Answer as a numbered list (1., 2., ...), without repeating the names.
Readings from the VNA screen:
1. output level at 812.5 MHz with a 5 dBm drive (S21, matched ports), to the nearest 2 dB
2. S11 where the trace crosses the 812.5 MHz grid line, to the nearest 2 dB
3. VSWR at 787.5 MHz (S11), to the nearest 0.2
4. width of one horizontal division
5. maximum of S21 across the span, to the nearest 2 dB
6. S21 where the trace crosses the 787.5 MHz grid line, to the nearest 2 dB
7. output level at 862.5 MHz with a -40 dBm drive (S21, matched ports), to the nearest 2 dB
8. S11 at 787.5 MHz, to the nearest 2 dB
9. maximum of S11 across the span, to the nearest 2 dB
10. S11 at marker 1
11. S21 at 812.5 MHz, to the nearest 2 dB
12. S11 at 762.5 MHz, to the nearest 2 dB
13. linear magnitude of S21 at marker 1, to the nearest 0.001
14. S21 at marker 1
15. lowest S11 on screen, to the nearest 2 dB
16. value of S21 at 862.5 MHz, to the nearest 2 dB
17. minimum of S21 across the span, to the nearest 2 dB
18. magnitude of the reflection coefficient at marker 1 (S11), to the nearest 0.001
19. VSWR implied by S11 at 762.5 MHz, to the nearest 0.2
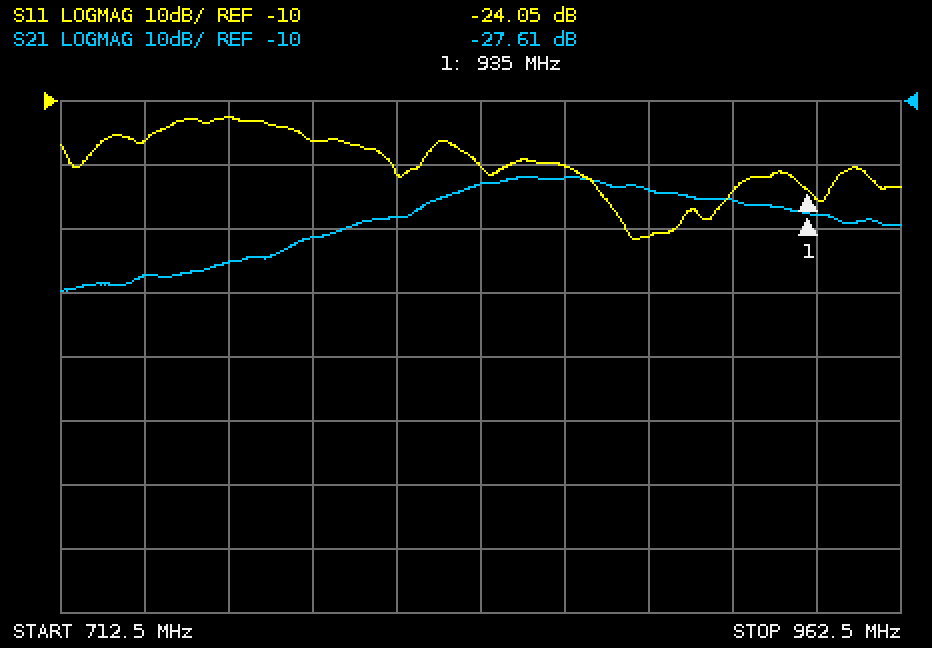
1. -24 dBm
2. -22 dB
3. 1.4
4. 25 MHz
5. -22 dB
6. -32 dB
7. -62 dBm
8. -16 dB
9. -12 dB
10. -24.05 dB
11. -28 dB
12. -12 dB
13. 0.042
14. -27.61 dB
15. -32 dB
16. -22 dB
17. -40 dB
18. 0.063
19. 1.6
